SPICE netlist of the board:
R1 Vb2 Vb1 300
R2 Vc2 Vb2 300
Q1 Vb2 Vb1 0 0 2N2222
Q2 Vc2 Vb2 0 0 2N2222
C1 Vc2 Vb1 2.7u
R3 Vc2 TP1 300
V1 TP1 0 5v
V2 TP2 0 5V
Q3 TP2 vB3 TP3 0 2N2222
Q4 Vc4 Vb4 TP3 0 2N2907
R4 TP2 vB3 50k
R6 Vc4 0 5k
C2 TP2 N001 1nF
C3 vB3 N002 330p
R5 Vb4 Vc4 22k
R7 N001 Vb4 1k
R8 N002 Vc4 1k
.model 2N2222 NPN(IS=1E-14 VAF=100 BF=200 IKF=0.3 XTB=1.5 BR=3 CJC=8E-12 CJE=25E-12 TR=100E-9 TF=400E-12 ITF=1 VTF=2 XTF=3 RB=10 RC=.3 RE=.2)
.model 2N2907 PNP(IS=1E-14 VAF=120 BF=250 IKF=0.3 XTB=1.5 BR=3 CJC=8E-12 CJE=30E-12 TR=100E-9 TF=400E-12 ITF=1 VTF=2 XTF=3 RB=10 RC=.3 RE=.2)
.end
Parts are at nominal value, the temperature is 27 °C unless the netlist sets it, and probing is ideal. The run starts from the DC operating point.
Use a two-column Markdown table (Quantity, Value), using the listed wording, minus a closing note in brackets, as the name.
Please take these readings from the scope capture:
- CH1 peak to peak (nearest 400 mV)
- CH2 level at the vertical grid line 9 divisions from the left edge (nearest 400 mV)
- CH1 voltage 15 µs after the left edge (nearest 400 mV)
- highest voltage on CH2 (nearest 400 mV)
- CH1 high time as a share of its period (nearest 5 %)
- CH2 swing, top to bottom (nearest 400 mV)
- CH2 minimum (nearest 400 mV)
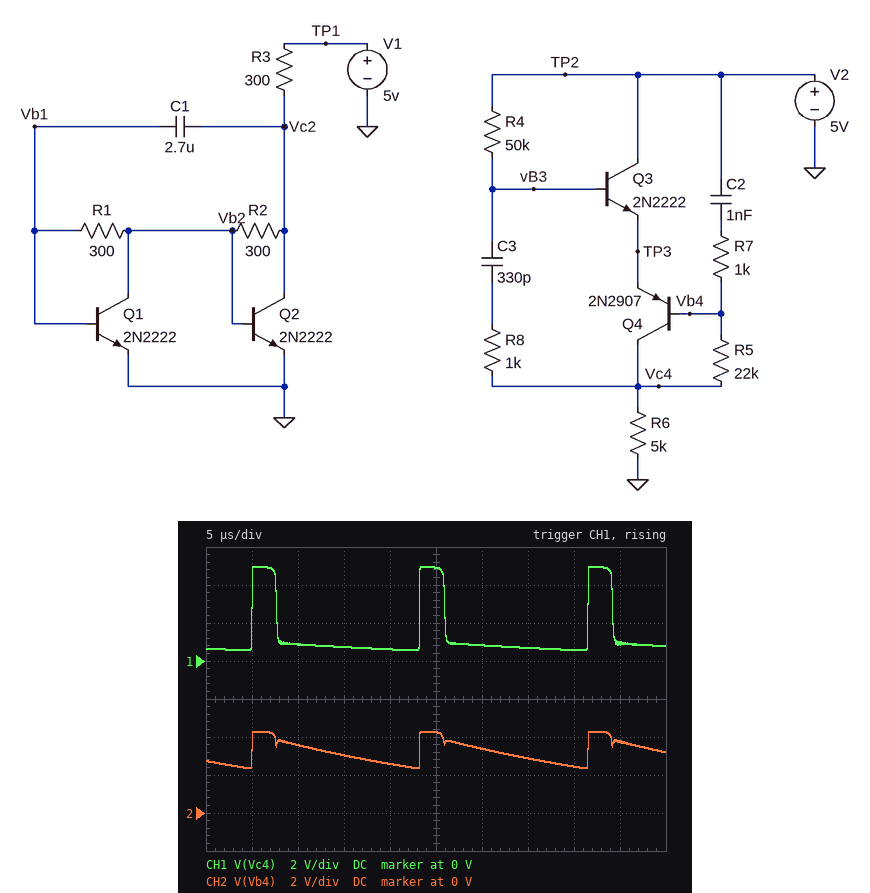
| Quantity | Value |
|---|---|
| CH1 peak to peak | 4.4 V |
| CH2 level at the vertical grid line 9 divisions from the left edge | 3.6 V |
| CH1 voltage 15 µs after the left edge | 800 mV |
| highest voltage on CH2 | 4.4 V |
| CH1 high time as a share of its period | 15 % |
| CH2 swing, top to bottom | 2.0 V |
| CH2 minimum | 2.4 V |
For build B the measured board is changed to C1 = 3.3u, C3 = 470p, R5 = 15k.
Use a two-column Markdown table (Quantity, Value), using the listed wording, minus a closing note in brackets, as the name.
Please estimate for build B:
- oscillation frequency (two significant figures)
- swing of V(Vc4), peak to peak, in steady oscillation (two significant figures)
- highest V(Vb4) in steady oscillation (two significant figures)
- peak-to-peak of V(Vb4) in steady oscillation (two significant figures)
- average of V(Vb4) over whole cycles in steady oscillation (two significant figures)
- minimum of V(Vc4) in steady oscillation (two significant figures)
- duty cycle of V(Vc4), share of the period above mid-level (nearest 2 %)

| Quantity | Value |
|---|---|
| oscillation frequency | 52 kHz |
| swing of V(Vc4), peak to peak, in steady oscillation | 4.3 V |
| highest V(Vb4) in steady oscillation | 4.3 V |
| peak-to-peak of V(Vb4) in steady oscillation | 2.3 V |
| average of V(Vb4) over whole cycles in steady oscillation | 3.0 V |
| minimum of V(Vc4) in steady oscillation | 650 mV |
| duty cycle of V(Vc4), share of the period above mid-level | 16 % |
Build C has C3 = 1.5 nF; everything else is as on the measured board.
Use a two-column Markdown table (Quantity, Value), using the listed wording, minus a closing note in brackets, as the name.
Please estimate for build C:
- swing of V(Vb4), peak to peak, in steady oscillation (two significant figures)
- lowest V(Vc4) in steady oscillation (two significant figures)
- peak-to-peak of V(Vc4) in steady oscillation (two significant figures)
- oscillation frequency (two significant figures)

| Quantity | Value |
|---|---|
| swing of V(Vb4), peak to peak, in steady oscillation | 2.8 V |
| lowest V(Vc4) in steady oscillation | 490 mV |
| peak-to-peak of V(Vc4) in steady oscillation | 4.5 V |
| oscillation frequency | 26 kHz |
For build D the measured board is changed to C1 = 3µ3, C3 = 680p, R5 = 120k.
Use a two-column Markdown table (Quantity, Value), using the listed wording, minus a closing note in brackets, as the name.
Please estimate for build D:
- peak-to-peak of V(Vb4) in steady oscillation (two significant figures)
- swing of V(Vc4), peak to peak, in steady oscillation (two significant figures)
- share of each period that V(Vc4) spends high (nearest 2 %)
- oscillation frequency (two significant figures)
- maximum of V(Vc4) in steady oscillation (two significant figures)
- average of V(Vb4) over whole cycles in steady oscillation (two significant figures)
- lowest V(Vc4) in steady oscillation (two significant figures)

| Quantity | Value |
|---|---|
| peak-to-peak of V(Vb4) in steady oscillation | 1.4 V |
| swing of V(Vc4), peak to peak, in steady oscillation | 4.7 V |
| share of each period that V(Vc4) spends high | 8 % |
| oscillation frequency | 19 kHz |
| maximum of V(Vc4) in steady oscillation | 5.0 V |
| average of V(Vb4) over whole cycles in steady oscillation | 3.5 V |
| lowest V(Vc4) in steady oscillation | 220 mV |
